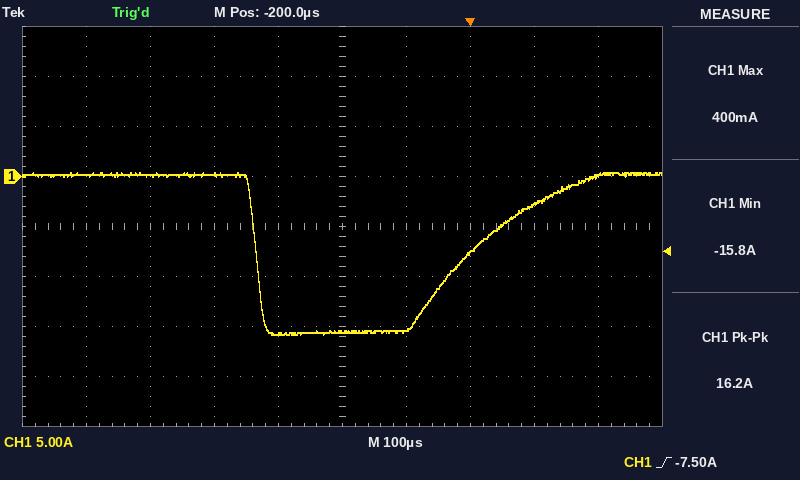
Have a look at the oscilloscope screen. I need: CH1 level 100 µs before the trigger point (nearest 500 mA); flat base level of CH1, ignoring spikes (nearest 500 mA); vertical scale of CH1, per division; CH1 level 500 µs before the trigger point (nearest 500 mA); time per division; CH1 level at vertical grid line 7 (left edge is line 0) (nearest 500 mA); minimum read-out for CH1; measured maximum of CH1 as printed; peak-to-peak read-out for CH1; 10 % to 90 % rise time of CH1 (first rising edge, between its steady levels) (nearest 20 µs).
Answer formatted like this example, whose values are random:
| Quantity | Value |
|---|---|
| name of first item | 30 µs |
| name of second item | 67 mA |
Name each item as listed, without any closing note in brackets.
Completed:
| Quantity | Value |
|---|---|
| CH1 level 100 µs before the trigger point | -15.5 A |
| flat base level of CH1, ignoring spikes | -15.5 A |
| vertical scale of CH1, per division | 5 A |
| CH1 level 500 µs before the trigger point | 0.0 A |
| time per division | 100 µs |
| CH1 level at vertical grid line 7 (left edge is line 0) | -7.5 A |
| minimum read-out for CH1 | -15.8 A |
| measured maximum of CH1 as printed | 400 mA |
| peak-to-peak read-out for CH1 | 16.2 A |
| 10 % to 90 % rise time of CH1 (first rising edge, between its steady levels) | 220 µs |
